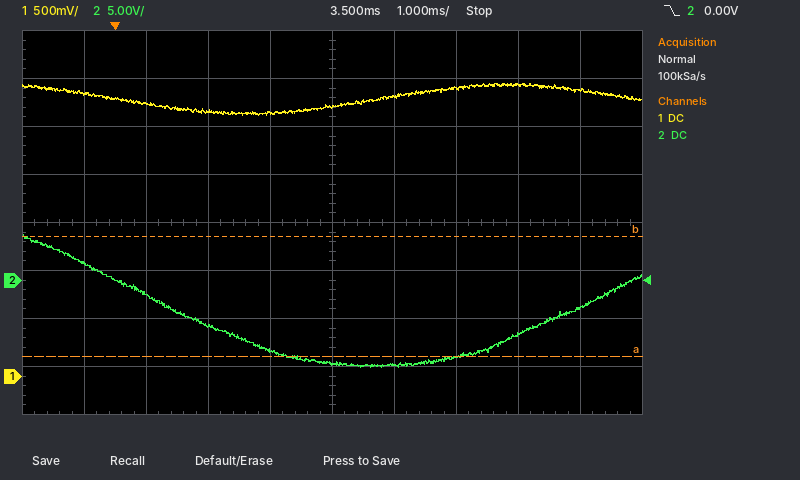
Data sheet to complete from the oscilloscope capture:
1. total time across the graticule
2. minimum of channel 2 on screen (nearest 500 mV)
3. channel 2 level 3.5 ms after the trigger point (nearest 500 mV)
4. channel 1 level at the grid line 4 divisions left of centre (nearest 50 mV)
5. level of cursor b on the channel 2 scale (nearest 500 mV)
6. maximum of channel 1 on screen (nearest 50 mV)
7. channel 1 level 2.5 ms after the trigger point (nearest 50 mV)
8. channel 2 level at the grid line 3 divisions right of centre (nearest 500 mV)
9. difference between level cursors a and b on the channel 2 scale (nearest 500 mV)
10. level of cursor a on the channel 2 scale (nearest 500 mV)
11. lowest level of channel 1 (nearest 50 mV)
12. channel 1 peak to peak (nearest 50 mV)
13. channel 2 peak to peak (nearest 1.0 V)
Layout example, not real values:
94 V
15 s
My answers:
10 ms
-9.0 V
-8.5 V
2.95 V
4.5 V
3.05 V
2.75 V
-5.5 V
12.5 V
-8.0 V
2.70 V
350 mV
14.0 V
